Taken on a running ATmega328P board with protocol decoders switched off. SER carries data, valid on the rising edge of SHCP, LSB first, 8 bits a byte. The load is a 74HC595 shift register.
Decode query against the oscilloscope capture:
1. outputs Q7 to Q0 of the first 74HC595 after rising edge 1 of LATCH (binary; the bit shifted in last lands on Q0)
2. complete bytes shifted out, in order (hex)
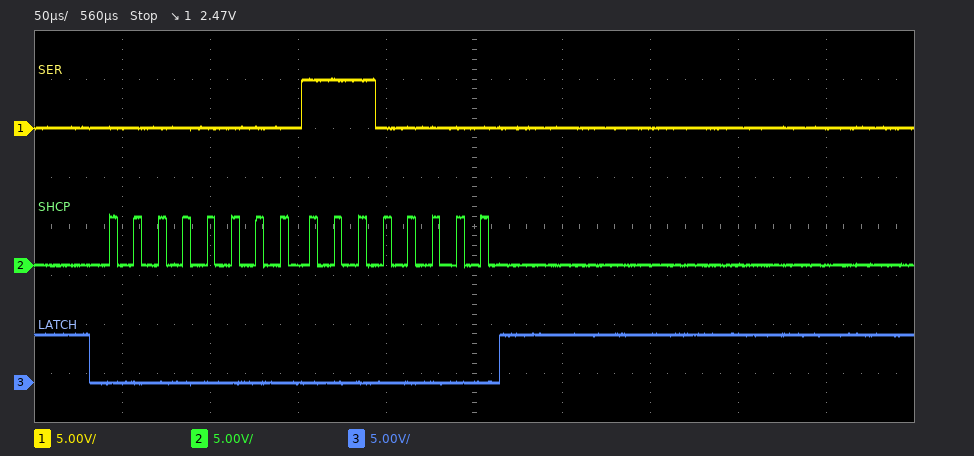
11100000
00 07
